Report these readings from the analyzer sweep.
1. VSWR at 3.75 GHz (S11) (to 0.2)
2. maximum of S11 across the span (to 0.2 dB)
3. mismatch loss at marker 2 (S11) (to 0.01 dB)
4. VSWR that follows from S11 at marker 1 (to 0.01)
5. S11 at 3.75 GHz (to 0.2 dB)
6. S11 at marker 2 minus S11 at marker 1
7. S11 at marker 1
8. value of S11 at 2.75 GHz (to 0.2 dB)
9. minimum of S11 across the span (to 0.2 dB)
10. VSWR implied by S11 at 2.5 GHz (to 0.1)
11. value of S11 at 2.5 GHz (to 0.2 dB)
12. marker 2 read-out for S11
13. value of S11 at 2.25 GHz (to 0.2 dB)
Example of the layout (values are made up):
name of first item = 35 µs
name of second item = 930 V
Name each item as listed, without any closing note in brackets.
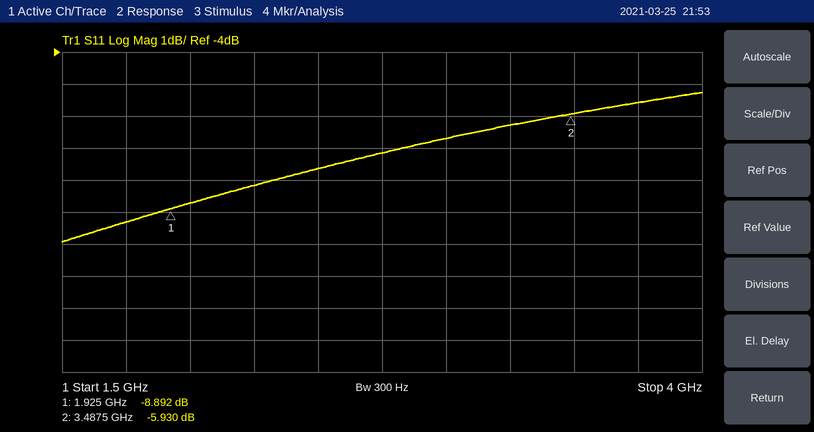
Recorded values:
VSWR at 3.75 GHz (S11) = 3.2
maximum of S11 across the span = -5.2 dB
mismatch loss at marker 2 (S11) = 1.28 dB
VSWR that follows from S11 at marker 1 = 2.12
S11 at 3.75 GHz = -5.6 dB
S11 at marker 2 minus S11 at marker 1 = 2.962 dB
S11 at marker 1 = -8.892 dB
value of S11 at 2.75 GHz = -7.2 dB
minimum of S11 across the span = -10.0 dB
VSWR implied by S11 at 2.5 GHz = 2.4
value of S11 at 2.5 GHz = -7.6 dB
marker 2 read-out for S11 = -5.930 dB
value of S11 at 2.25 GHz = -8.2 dB
